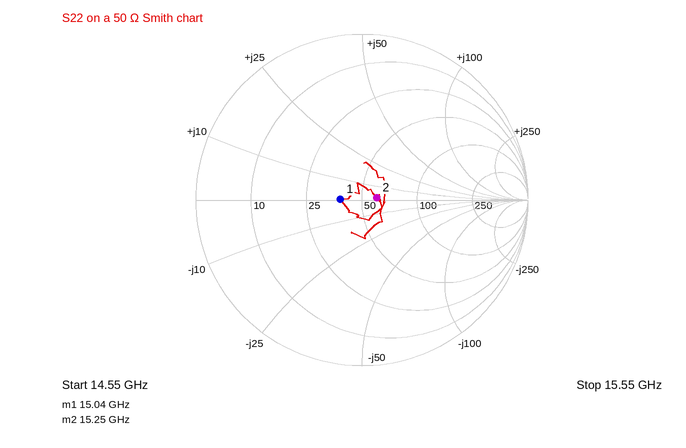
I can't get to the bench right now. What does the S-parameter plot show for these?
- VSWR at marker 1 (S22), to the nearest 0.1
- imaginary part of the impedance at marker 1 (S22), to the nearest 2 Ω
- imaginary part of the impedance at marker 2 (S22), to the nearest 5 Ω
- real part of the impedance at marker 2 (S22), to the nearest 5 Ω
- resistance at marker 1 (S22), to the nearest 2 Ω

1.3
0 Ω
0 Ω
60 Ω
38 Ω
